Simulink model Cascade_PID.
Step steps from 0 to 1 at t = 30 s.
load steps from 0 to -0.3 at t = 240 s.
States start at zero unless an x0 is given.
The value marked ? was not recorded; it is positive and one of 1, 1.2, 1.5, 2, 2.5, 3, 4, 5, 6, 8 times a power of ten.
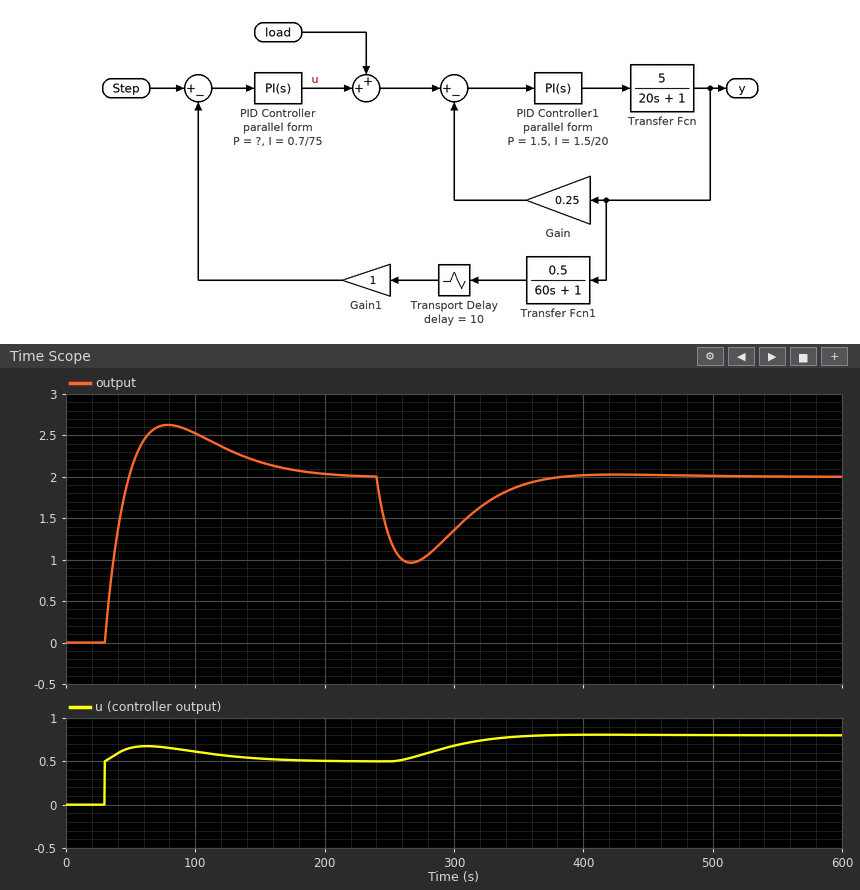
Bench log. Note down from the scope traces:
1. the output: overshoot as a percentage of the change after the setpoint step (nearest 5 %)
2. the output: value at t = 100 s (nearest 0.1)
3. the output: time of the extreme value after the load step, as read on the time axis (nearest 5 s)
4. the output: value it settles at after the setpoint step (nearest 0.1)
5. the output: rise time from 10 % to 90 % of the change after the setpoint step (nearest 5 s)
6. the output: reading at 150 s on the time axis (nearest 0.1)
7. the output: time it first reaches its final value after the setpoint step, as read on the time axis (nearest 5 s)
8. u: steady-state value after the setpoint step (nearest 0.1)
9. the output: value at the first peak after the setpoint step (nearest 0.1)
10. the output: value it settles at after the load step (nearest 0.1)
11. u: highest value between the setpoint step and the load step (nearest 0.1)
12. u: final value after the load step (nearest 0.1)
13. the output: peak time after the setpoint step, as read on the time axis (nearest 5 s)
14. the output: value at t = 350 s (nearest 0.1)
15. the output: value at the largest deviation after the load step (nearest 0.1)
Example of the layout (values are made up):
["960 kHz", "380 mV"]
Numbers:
["30 %", "2.5", "265 s", "2.0", "15 s", "2.2", "50 s", "0.5", "2.6", "2.0", "0.7", "0.8", "80 s", "1.9", "1.0"]
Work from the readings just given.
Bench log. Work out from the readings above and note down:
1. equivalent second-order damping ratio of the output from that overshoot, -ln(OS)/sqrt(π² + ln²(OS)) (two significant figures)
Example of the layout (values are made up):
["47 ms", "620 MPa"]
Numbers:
["0.36"]
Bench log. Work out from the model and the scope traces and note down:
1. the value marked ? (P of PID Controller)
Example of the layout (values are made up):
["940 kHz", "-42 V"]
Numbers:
["0.5"]
